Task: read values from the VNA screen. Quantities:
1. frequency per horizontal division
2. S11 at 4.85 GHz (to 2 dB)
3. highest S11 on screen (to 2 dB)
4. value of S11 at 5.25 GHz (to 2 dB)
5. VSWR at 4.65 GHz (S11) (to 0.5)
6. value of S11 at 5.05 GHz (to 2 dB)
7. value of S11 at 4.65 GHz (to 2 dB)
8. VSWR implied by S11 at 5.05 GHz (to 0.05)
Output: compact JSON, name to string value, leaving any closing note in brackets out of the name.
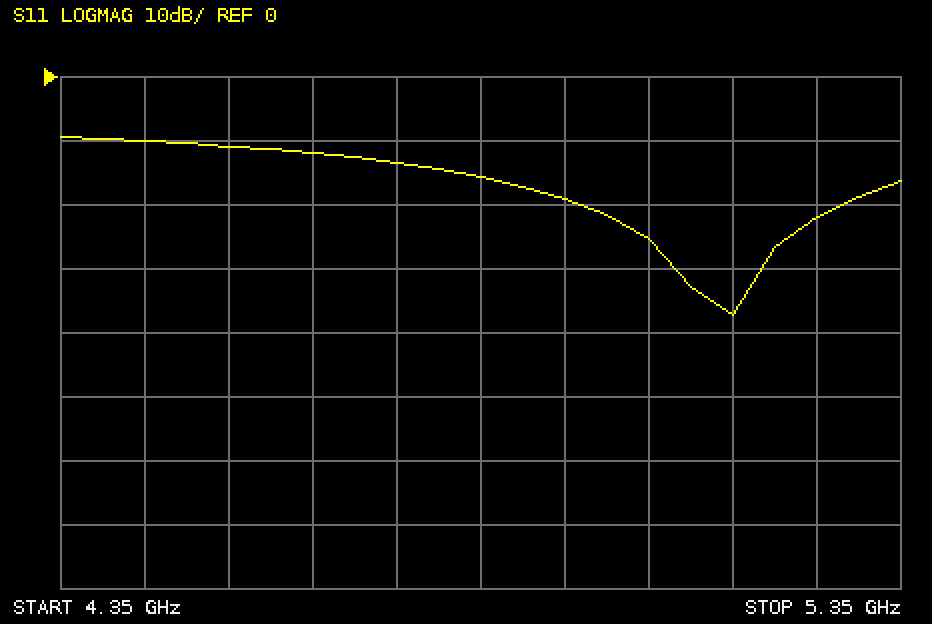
{"frequency per horizontal division": "100 MHz", "S11 at 4.85 GHz": "-16 dB", "highest S11 on screen": "-10 dB", "value of S11 at 5.25 GHz": "-22 dB", "VSWR at 4.65 GHz (S11)": "1.5", "value of S11 at 5.05 GHz": "-26 dB", "value of S11 at 4.65 GHz": "-12 dB", "VSWR implied by S11 at 5.05 GHz": "1.10"}
